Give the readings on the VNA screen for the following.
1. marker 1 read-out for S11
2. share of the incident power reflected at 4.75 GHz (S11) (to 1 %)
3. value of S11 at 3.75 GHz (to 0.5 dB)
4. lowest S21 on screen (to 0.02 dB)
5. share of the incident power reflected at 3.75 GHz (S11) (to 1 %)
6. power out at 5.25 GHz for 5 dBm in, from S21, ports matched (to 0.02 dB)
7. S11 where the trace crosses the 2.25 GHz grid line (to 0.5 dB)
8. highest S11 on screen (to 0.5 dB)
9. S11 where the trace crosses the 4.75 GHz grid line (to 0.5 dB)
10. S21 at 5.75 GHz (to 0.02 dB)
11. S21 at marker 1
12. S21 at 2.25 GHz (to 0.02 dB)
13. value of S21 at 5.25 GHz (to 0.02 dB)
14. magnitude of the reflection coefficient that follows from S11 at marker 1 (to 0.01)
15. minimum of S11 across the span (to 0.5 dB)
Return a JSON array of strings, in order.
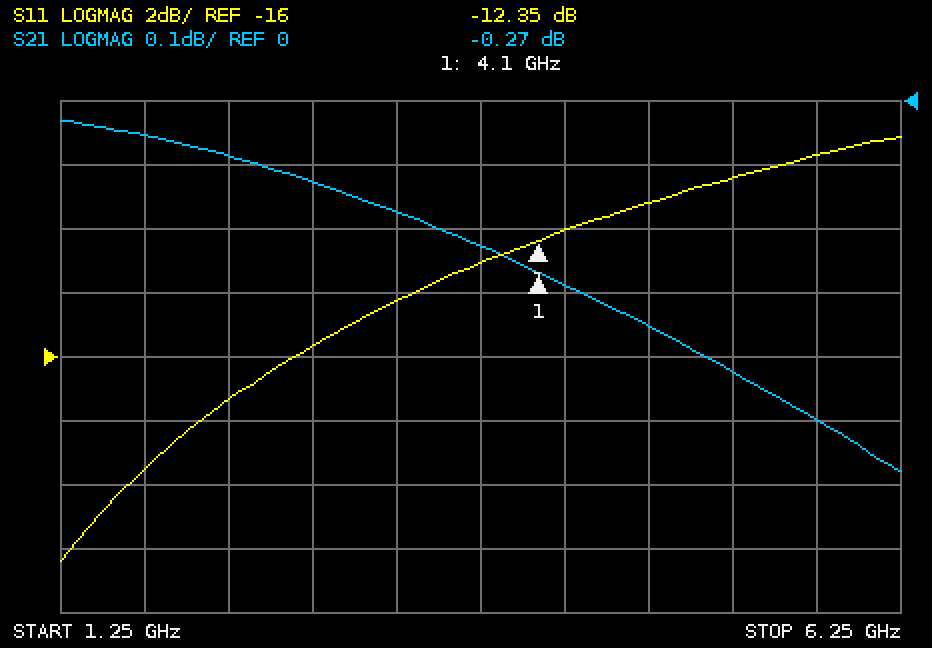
["-12.35 dB", "8 %", "-13.0 dB", "-0.58 dB", "5 %", "4.58 dBm", "-17.5 dB", "-9.0 dB", "-11.0 dB", "-0.50 dB", "-0.27 dB", "-0.08 dB", "-0.42 dB", "0.24", "-22.5 dB"]
